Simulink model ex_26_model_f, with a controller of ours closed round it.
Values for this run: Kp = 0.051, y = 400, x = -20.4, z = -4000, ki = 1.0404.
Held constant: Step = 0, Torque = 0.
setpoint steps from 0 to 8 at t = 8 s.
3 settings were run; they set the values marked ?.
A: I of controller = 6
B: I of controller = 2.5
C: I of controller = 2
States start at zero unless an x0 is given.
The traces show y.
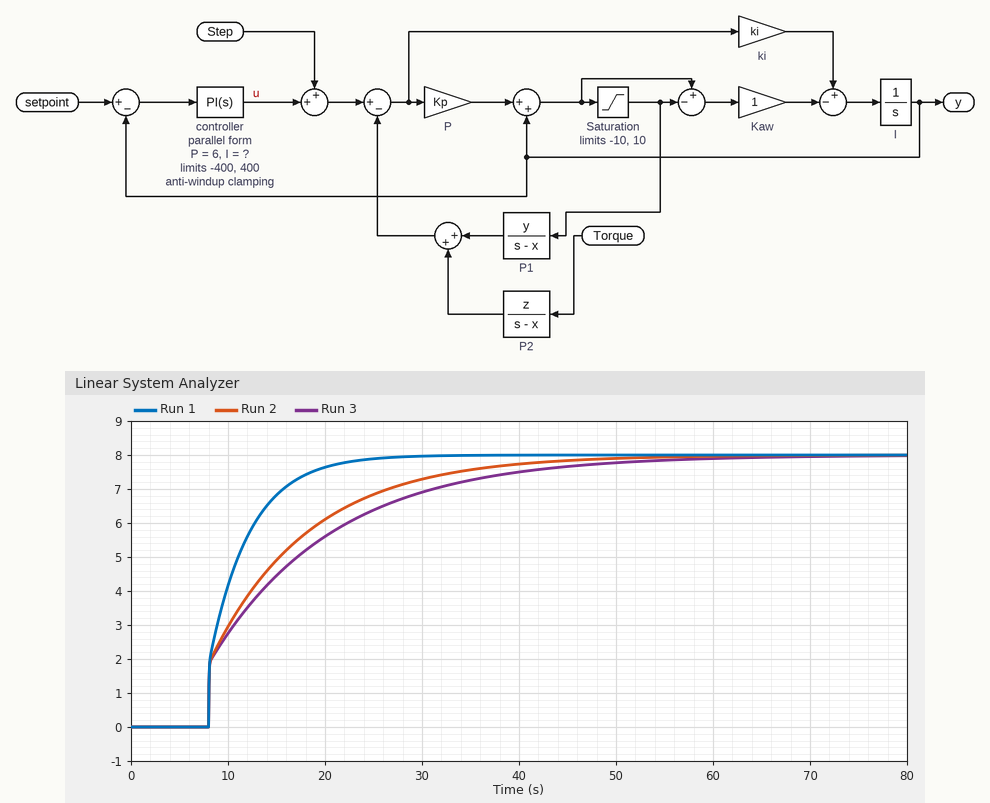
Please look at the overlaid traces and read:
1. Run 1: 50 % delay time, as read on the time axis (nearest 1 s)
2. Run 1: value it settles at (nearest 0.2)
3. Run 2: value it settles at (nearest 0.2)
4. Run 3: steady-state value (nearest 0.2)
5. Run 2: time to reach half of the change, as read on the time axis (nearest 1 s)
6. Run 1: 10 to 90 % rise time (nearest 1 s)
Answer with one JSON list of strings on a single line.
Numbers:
["10 s", "8.0", "8.0", "8.0", "12 s", "9 s"]
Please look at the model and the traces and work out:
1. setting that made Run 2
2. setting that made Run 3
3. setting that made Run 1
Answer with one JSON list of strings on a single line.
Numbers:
["B", "C", "A"]
